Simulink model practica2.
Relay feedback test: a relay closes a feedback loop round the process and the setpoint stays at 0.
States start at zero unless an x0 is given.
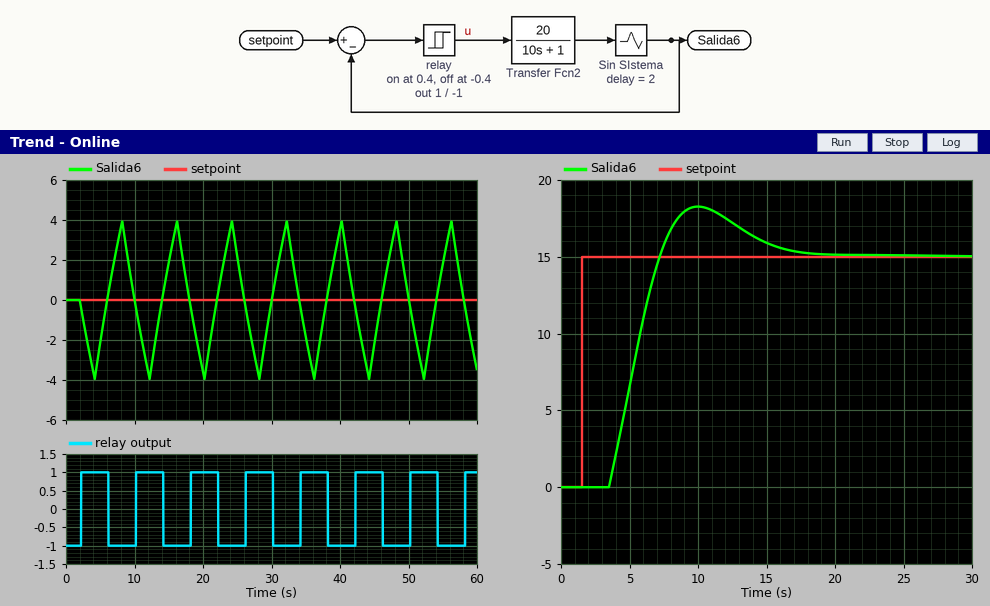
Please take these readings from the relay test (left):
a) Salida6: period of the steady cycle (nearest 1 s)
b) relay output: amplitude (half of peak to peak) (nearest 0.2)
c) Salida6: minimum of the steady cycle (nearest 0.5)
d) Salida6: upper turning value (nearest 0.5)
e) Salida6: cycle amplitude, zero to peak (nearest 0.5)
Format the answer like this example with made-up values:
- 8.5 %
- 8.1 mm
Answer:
- 8 s
- 1.0
- -4.0
- 4.0
- 4.0
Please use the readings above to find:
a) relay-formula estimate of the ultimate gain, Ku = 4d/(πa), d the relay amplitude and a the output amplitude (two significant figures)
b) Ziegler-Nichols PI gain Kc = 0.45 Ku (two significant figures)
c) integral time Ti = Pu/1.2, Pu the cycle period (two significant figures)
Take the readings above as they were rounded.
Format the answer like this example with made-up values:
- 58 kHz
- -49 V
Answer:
- 0.32
- 0.14
- 6.7 s
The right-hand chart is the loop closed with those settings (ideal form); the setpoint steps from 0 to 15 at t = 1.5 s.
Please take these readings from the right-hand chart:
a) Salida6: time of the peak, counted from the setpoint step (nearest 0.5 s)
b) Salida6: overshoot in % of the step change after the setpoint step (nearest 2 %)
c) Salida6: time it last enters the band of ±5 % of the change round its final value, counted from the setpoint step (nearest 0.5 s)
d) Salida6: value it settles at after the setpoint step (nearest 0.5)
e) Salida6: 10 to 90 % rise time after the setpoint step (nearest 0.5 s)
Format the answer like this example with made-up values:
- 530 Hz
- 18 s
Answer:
- 8.5 s
- 22 %
- 14.0 s
- 15.0
- 3.0 s
